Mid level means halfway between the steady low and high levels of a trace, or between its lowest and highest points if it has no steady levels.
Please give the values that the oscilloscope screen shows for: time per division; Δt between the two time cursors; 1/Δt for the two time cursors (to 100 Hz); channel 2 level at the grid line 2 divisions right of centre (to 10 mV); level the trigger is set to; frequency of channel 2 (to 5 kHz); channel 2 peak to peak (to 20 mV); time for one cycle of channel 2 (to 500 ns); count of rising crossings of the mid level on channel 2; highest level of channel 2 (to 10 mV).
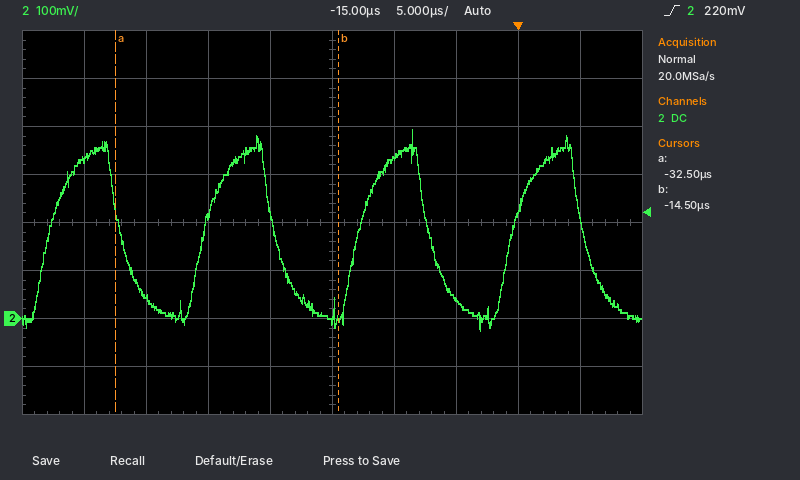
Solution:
5 µs
18.0 µs
55.6 kHz
40 mV
220 mV
80 kHz
420 mV
12.5 µs
4
390 mV
